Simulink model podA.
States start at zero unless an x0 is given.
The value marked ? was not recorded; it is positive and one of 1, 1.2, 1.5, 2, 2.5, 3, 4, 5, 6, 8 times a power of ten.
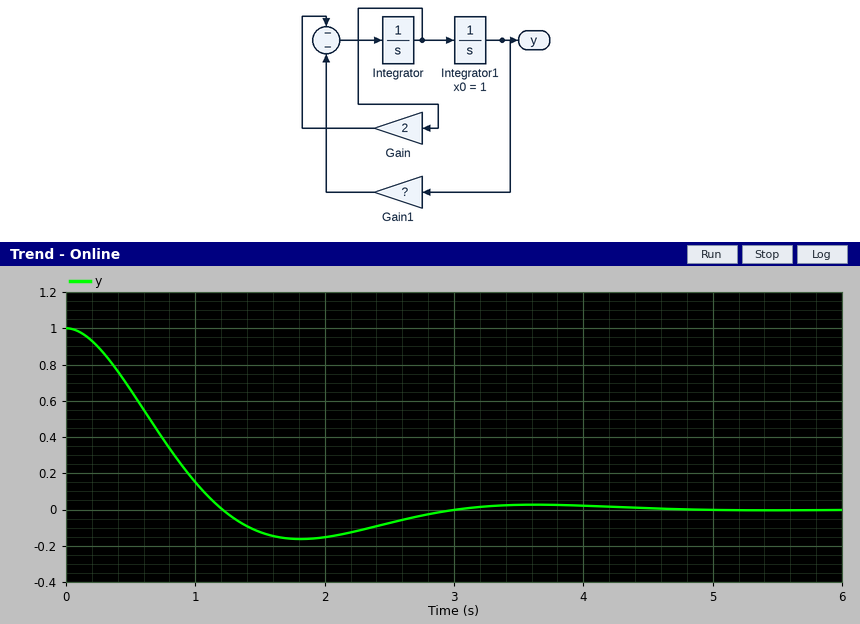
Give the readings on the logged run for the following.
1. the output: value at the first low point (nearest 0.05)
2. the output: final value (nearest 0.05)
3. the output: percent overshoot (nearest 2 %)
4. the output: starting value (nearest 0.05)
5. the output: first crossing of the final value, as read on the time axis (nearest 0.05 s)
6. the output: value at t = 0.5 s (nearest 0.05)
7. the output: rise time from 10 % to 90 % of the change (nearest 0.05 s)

-0.15
0.00
16 %
1.00
1.20 s
0.65
0.80 s
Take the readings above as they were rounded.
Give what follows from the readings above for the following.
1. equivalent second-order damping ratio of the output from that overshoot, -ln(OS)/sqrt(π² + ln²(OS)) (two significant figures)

0.50
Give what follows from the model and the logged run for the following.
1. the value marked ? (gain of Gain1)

4
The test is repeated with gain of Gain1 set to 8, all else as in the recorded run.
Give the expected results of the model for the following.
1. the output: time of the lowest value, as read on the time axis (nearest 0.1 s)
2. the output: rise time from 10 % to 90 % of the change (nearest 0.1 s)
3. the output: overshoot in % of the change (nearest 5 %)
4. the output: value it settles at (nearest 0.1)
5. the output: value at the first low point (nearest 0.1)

1.2 s
0.5 s
30 %
0.0
-0.3
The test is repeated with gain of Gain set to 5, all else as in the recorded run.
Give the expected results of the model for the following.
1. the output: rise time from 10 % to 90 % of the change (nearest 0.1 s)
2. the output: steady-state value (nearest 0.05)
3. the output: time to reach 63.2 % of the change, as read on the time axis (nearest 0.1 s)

2.3 s
0.00
1.3 s
